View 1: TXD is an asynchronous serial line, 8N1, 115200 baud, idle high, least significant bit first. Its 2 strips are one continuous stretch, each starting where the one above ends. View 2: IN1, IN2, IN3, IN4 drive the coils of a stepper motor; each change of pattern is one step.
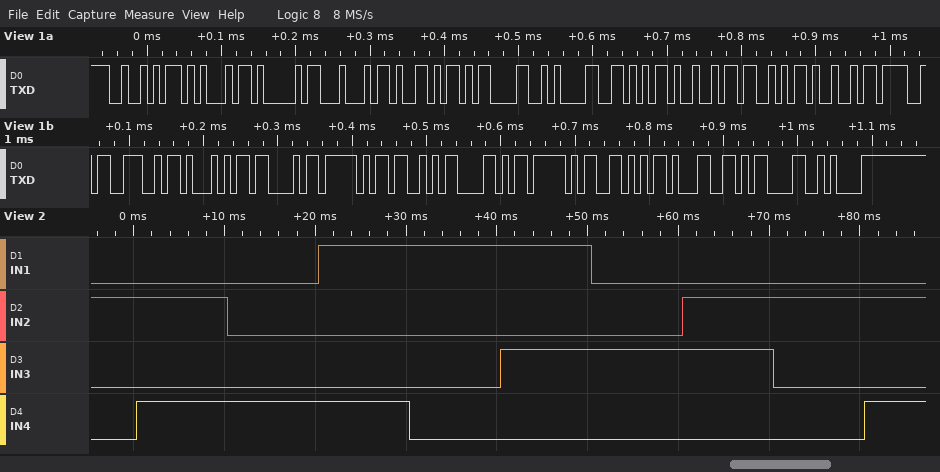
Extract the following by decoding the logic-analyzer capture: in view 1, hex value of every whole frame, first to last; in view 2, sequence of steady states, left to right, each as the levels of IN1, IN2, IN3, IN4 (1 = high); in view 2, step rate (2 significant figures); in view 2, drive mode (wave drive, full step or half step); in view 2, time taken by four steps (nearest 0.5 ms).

0x52 0x45 0x41 0x44 0x59 0x0D 0x0A 0x56 0x49 0x53 0x49 0x4F 0x4E 0x51 0x43 0x5F 0x53 0x58 0x5F 0x56 0x31 0x0D 0x0A
0100 0101 0001 1001 1000 1010 0010 0110 0100 0101
100 steps/s
half step
40.0 ms
